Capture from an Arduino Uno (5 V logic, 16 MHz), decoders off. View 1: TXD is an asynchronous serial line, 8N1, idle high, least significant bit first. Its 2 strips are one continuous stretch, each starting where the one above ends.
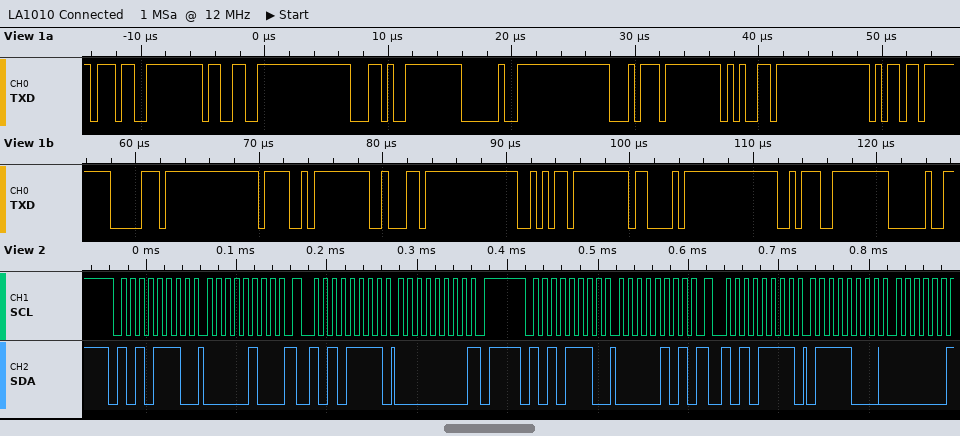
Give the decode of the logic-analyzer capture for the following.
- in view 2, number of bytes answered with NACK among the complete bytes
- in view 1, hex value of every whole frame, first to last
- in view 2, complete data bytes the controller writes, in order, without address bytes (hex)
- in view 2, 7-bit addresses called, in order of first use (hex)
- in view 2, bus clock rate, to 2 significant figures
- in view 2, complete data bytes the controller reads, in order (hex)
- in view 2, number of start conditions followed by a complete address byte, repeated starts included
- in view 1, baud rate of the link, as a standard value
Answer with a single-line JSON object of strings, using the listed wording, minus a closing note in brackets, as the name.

{"in view 2, number of bytes answered with NACK among the complete bytes": "1", "in view 1, hex value of every whole frame, first to last": "37 33 2C 20 74 65 6D 70 4F 62 6A 43 3A 20", "in view 2, complete data bytes the controller writes, in order, without address bytes": "04 05", "in view 2, 7-bit addresses called, in order of first use": "0x57", "in view 2, bus clock rate, to 2 significant figures": "100 kHz", "in view 2, complete data bytes the controller reads, in order": "00 78", "in view 2, number of start conditions followed by a complete address byte, repeated starts included": "4", "in view 1, baud rate of the link, as a standard value": "2000000 baud"}
